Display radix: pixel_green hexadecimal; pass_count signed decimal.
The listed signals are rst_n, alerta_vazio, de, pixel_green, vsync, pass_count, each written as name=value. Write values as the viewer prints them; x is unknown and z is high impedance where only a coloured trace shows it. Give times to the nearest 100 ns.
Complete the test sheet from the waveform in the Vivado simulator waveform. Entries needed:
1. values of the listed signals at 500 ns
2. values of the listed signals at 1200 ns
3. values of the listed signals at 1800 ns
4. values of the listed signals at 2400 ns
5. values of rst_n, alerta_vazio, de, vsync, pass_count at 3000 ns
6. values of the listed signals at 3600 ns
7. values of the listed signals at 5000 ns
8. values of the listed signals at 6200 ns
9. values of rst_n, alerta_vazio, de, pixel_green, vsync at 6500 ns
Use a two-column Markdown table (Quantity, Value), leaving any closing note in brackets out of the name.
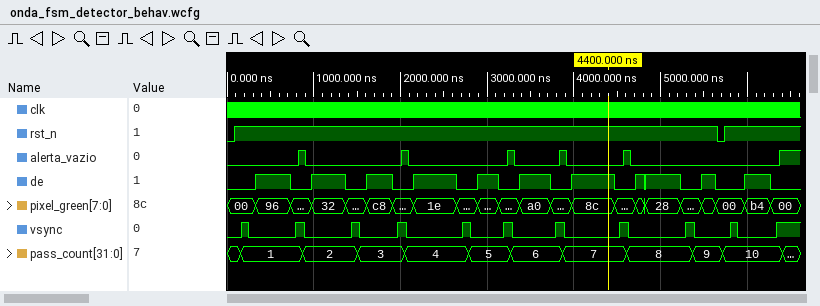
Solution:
| Quantity | Value |
|---|---|
| values of the listed signals at 500 ns | rst_n=1, alerta_vazio=0, de=1, pixel_green=96, vsync=0, pass_count=1 |
| values of the listed signals at 1200 ns | rst_n=1, alerta_vazio=0, de=1, pixel_green=32, vsync=0, pass_count=2 |
| values of the listed signals at 1800 ns | rst_n=1, alerta_vazio=0, de=1, pixel_green=c8, vsync=0, pass_count=3 |
| values of the listed signals at 2400 ns | rst_n=1, alerta_vazio=0, de=1, pixel_green=1e, vsync=0, pass_count=4 |
| values of rst_n, alerta_vazio, de, vsync, pass_count at 3000 ns | rst_n=1, alerta_vazio=0, de=1, vsync=0, pass_count=5 |
| values of the listed signals at 3600 ns | rst_n=1, alerta_vazio=0, de=1, pixel_green=a0, vsync=0, pass_count=6 |
| values of the listed signals at 5000 ns | rst_n=1, alerta_vazio=0, de=1, pixel_green=28, vsync=0, pass_count=8 |
| values of the listed signals at 6200 ns | rst_n=1, alerta_vazio=0, de=1, pixel_green=b4, vsync=0, pass_count=10 |
| values of rst_n, alerta_vazio, de, pixel_green, vsync at 6500 ns | rst_n=1, alerta_vazio=1, de=0, pixel_green=00, vsync=1 |
